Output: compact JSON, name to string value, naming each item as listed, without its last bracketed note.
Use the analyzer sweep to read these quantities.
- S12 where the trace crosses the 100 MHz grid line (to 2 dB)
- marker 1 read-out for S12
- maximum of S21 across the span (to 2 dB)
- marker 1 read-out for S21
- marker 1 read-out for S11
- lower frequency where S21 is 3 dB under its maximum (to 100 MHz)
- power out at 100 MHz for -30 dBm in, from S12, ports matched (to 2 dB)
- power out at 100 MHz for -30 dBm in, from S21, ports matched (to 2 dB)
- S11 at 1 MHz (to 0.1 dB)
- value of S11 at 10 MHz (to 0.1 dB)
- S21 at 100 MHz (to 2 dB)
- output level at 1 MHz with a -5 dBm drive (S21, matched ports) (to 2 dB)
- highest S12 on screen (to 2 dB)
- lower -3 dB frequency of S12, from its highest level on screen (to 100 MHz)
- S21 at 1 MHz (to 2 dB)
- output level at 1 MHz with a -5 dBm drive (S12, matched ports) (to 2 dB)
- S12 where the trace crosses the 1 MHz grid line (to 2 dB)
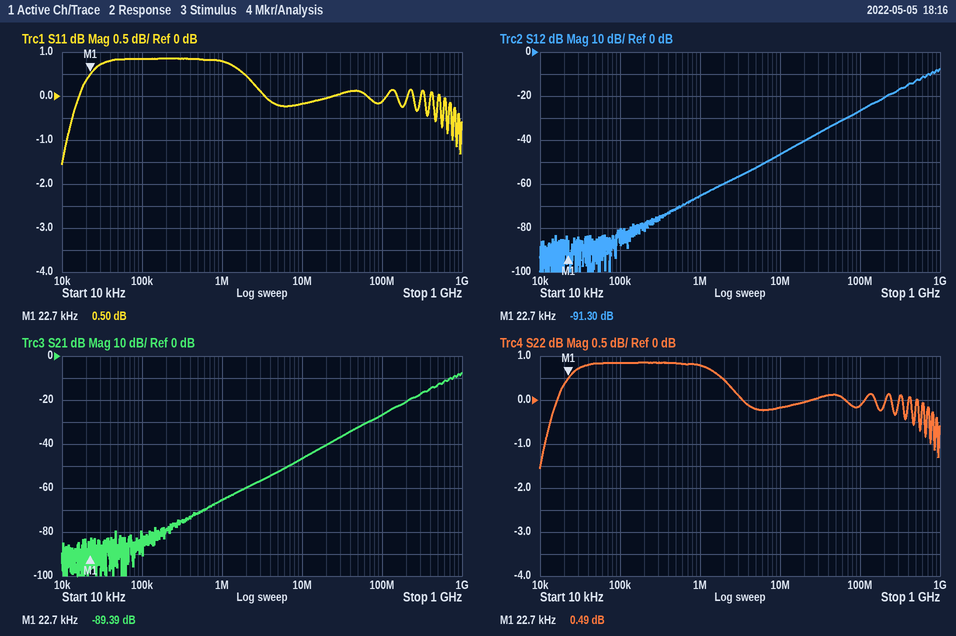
{"S12 where the trace crosses the 100 MHz grid line": "-26 dB", "marker 1 read-out for S12": "-91.30 dB", "maximum of S21 across the span": "-8 dB", "marker 1 read-out for S21": "-89.39 dB", "marker 1 read-out for S11": "0.50 dB", "lower frequency where S21 is 3 dB under its maximum": "700 MHz", "power out at 100 MHz for -30 dBm in, from S12, ports matched": "-56 dBm", "power out at 100 MHz for -30 dBm in, from S21, ports matched": "-56 dBm", "S11 at 1 MHz": "0.8 dB", "value of S11 at 10 MHz": "-0.2 dB", "S21 at 100 MHz": "-26 dB", "output level at 1 MHz with a -5 dBm drive (S21, matched ports)": "-70 dBm", "highest S12 on screen": "-8 dB", "lower -3 dB frequency of S12, from its highest level on screen": "700 MHz", "S21 at 1 MHz": "-66 dB", "output level at 1 MHz with a -5 dBm drive (S12, matched ports)": "-70 dBm", "S12 where the trace crosses the 1 MHz grid line": "-66 dB"}
